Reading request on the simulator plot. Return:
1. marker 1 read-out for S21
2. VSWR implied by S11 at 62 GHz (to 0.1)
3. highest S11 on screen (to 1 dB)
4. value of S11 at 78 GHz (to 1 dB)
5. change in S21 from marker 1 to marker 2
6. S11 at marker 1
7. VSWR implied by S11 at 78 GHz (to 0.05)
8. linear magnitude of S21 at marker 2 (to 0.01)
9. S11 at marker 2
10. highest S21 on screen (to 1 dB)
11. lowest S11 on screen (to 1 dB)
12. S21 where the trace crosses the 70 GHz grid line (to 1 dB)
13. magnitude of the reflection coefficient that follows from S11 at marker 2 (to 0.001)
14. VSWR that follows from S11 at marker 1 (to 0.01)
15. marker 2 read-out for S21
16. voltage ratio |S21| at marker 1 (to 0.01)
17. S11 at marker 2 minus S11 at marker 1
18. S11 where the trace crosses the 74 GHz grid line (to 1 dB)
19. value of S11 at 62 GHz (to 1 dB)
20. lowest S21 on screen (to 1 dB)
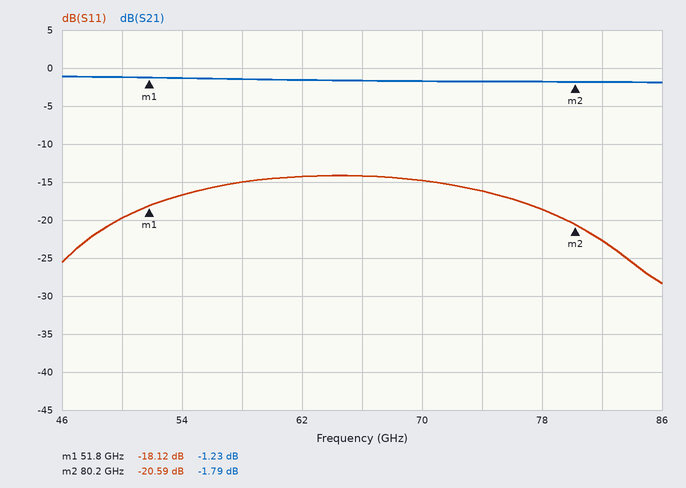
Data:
-1.23 dB
1.5
-14 dB
-19 dB
-0.56 dB
-18.12 dB
1.25
0.81
-20.59 dB
-1 dB
-28 dB
-2 dB
0.093
1.28
-1.79 dB
0.87
-2.47 dB
-16 dB
-14 dB
-2 dB
